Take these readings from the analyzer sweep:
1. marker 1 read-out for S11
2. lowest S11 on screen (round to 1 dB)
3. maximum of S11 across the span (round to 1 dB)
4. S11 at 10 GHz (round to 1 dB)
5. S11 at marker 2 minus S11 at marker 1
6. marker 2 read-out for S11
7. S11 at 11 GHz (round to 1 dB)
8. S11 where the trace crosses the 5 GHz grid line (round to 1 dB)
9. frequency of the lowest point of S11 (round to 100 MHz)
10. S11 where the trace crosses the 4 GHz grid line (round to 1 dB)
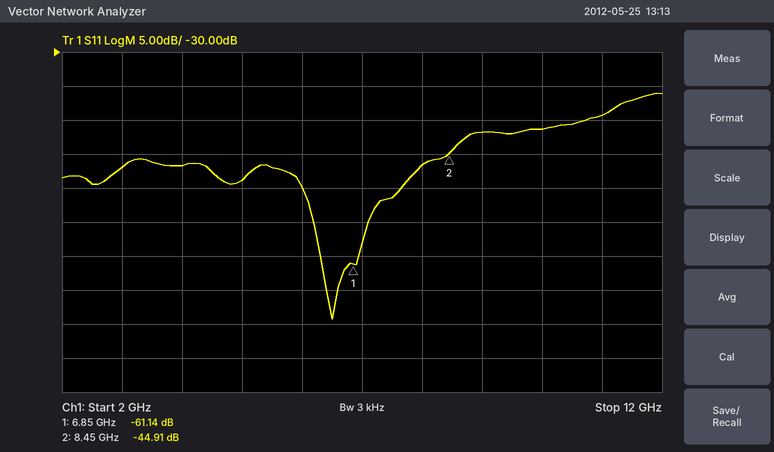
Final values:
-61.14 dB
-69 dB
-36 dB
-41 dB
16.23 dB
-44.91 dB
-39 dB
-49 dB
6.5 GHz
-47 dB
